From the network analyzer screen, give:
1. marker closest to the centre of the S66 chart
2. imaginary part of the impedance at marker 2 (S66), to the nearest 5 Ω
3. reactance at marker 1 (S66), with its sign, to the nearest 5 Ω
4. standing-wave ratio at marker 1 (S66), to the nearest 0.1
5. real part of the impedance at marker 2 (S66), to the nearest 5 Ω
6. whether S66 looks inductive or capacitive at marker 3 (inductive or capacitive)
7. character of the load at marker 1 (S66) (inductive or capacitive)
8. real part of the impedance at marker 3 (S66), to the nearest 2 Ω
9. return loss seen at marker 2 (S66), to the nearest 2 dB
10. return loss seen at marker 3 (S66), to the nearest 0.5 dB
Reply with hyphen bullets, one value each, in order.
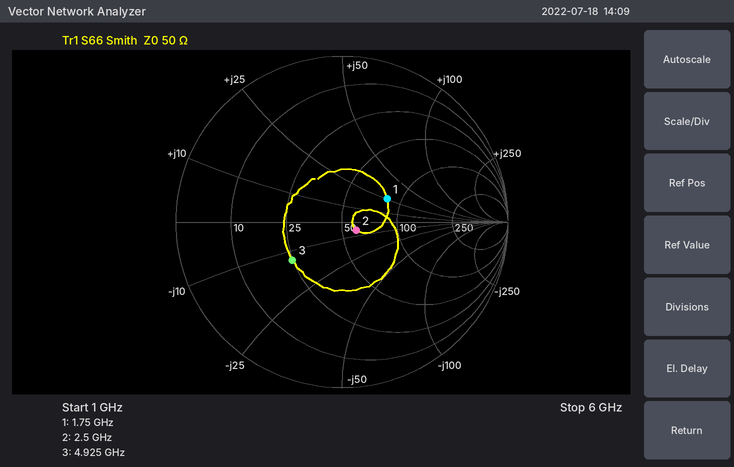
- marker 2
- -5 Ω
- +25 Ω
- 1.9
- 60 Ω
- capacitive
- inductive
- 24 Ω
- 20 dB
- 8.5 dB
